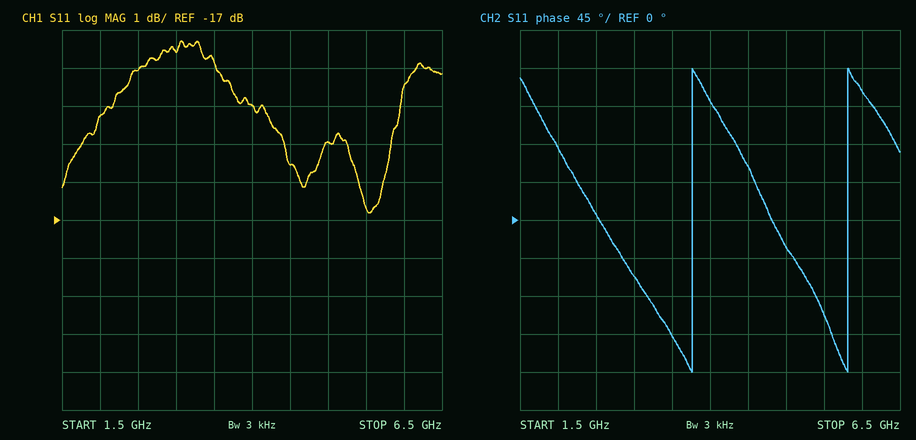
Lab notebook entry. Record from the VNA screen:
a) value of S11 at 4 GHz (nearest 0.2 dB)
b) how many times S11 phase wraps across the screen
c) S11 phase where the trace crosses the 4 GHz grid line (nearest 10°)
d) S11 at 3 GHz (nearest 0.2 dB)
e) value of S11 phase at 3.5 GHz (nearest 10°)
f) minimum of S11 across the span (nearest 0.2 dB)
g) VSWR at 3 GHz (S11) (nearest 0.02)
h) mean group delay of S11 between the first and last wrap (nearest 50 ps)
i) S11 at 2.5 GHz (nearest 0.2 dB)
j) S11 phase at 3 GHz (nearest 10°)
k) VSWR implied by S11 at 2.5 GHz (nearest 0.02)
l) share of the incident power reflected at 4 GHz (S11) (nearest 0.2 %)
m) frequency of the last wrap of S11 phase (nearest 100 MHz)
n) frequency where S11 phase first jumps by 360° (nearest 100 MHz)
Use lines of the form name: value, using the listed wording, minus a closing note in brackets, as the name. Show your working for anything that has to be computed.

value of S11 at 4 GHz: -14.0 dB
how many times S11 phase wraps across the screen: 2
S11 phase where the trace crosses the 4 GHz grid line: 140°
S11 at 3 GHz: -12.6 dB
value of S11 phase at 3.5 GHz: -140°
minimum of S11 across the span: -16.8 dB
VSWR at 3 GHz (S11): |Γ| = 10^(-12.6/20) = 0.2344; VSWR = (1 + 0.2344)/(1 − 0.2344) ≈ 1.61, so 1.62 to the nearest 0.02
mean group delay of S11 between the first and last wrap: 1 cycle / (5.8 GHz − 3.8 GHz) ≈ 500 ps
S11 at 2.5 GHz: -13.0 dB
S11 phase at 3 GHz: -70°
VSWR implied by S11 at 2.5 GHz: |Γ| = 10^(-13/20) = 0.2239; VSWR = (1 + 0.2239)/(1 − 0.2239) ≈ 1.58
share of the incident power reflected at 4 GHz (S11): 10^(-14/10) ≈ 4.0 %
frequency of the last wrap of S11 phase: 5.8 GHz
frequency where S11 phase first jumps by 360°: 3.8 GHz
